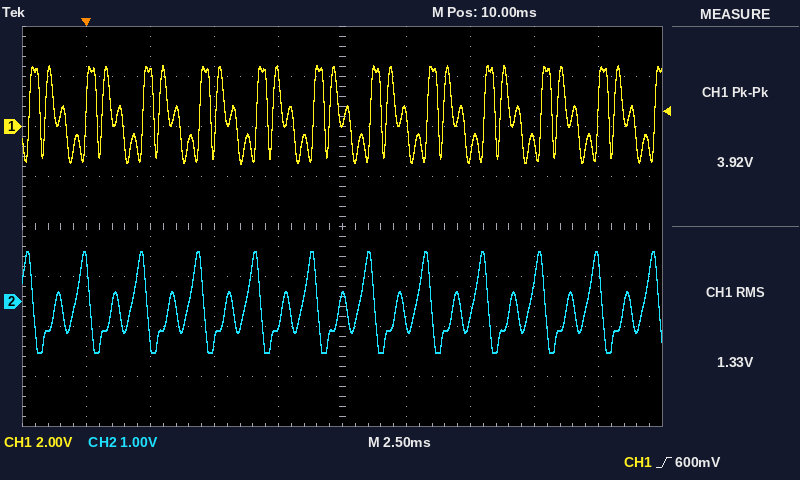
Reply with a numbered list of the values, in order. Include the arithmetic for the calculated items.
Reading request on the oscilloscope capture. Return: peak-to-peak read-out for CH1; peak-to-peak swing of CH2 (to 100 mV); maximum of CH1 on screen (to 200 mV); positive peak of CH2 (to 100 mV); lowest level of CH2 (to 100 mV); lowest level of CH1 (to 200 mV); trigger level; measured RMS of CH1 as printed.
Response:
1. 3.92 V
2. 1.0 V − (-1.0 V) = 2.0 V
3. 2.4 V
4. 1.0 V
5. -1.0 V
6. -1.4 V
7. 600 mV
8. 1.33 V
